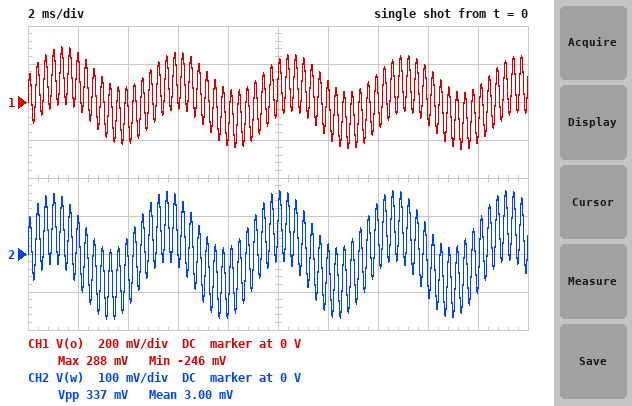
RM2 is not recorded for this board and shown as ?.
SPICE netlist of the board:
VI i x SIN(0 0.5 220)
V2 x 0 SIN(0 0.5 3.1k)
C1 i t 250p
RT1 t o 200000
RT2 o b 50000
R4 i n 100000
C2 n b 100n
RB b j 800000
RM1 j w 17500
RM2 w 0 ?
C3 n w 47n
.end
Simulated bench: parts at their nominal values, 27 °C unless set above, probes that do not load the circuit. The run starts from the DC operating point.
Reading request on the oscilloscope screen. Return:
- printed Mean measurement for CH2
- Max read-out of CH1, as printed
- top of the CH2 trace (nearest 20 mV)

3.00 mV
288 mV
160 mV
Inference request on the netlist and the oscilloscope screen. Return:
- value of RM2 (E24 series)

18 kΩ
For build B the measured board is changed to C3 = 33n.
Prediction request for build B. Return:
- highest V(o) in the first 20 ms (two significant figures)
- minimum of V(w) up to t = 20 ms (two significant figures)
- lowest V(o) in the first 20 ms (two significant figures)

310 mV
-170 mV
-260 mV
